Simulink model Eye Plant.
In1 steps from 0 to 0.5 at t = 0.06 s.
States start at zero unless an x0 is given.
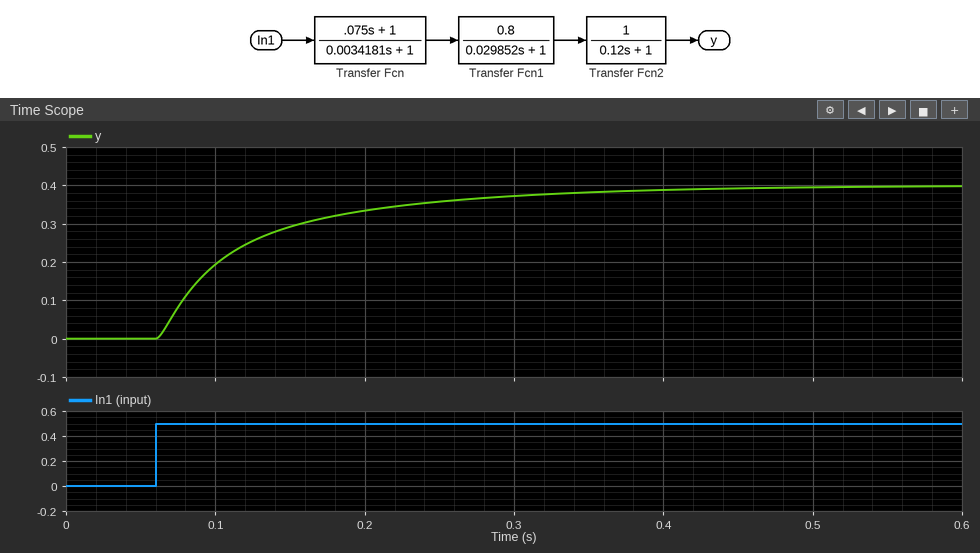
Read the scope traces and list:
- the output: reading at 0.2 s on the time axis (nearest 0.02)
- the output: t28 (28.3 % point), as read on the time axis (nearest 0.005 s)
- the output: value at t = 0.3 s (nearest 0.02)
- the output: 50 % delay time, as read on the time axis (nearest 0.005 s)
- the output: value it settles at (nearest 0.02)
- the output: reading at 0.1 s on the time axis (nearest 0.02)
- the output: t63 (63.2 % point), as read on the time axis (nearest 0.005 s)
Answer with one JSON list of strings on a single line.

["0.34", "0.080 s", "0.38", "0.100 s", "0.40", "0.20", "0.125 s"]
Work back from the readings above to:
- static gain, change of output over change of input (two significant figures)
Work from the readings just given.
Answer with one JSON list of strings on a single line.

["0.80"]
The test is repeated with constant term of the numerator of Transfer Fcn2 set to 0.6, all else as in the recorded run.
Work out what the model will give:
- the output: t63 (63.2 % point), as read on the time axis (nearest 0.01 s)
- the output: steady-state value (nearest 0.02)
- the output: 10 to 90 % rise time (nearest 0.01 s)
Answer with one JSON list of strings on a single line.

["0.12 s", "0.24", "0.19 s"]
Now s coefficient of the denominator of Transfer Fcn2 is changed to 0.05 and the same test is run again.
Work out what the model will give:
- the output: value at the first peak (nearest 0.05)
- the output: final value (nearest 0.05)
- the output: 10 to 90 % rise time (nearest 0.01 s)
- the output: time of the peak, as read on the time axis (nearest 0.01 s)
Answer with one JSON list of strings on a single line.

["0.45", "0.40", "0.03 s", "0.15 s"]
